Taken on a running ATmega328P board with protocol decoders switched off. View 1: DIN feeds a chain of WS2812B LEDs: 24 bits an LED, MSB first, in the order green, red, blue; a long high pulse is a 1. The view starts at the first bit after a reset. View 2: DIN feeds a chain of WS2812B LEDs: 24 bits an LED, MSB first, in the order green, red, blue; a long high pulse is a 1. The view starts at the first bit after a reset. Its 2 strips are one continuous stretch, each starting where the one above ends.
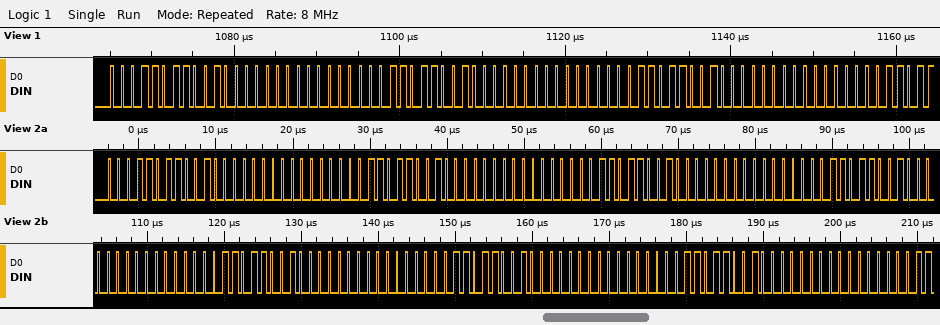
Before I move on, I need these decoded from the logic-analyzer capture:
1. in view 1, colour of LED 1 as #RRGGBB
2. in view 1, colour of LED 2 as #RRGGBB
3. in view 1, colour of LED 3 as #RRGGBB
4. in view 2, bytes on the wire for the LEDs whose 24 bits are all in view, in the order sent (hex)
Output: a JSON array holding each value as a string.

["#201B00", "#201B00", "#201B00", "1B 20 00 1B 20 00 1B 20 00 1B 20 00 1B 20 00 1B 20 00 1B 20 00"]
